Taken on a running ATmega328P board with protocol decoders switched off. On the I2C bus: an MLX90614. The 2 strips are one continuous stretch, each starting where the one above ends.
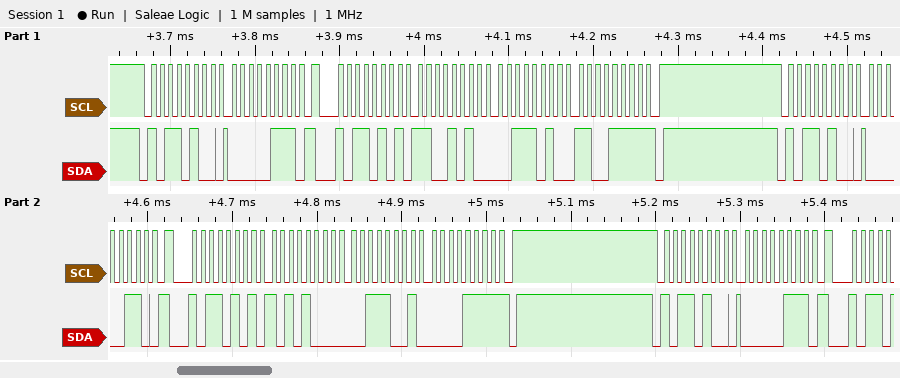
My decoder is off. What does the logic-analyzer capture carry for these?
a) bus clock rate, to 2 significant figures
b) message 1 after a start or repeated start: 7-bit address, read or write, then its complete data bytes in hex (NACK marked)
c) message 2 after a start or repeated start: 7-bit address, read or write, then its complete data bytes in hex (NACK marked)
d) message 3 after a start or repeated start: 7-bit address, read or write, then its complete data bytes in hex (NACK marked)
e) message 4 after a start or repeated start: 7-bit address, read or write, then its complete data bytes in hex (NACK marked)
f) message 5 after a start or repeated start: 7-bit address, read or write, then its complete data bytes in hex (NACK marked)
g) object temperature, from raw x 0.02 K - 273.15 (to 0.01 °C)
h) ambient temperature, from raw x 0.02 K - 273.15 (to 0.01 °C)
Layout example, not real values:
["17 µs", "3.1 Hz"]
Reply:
["100 kHz", "0x5A write: 07", "0x5A read: CA 3A CF NACK", "0x5A write: 06", "0x5A read: A8 39 0F NACK", "0x5A write: 07", "27.85 °C", "22.05 °C"]
